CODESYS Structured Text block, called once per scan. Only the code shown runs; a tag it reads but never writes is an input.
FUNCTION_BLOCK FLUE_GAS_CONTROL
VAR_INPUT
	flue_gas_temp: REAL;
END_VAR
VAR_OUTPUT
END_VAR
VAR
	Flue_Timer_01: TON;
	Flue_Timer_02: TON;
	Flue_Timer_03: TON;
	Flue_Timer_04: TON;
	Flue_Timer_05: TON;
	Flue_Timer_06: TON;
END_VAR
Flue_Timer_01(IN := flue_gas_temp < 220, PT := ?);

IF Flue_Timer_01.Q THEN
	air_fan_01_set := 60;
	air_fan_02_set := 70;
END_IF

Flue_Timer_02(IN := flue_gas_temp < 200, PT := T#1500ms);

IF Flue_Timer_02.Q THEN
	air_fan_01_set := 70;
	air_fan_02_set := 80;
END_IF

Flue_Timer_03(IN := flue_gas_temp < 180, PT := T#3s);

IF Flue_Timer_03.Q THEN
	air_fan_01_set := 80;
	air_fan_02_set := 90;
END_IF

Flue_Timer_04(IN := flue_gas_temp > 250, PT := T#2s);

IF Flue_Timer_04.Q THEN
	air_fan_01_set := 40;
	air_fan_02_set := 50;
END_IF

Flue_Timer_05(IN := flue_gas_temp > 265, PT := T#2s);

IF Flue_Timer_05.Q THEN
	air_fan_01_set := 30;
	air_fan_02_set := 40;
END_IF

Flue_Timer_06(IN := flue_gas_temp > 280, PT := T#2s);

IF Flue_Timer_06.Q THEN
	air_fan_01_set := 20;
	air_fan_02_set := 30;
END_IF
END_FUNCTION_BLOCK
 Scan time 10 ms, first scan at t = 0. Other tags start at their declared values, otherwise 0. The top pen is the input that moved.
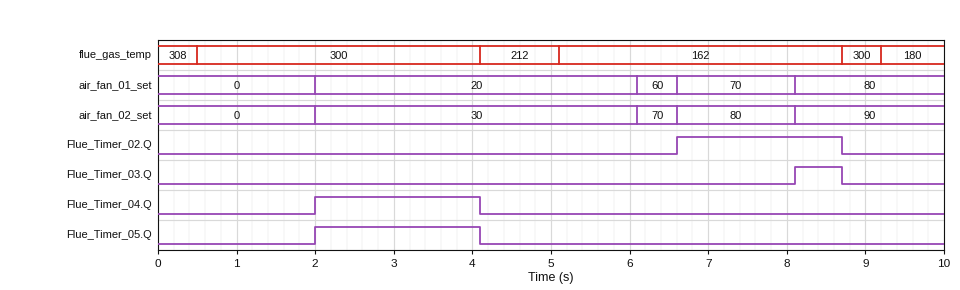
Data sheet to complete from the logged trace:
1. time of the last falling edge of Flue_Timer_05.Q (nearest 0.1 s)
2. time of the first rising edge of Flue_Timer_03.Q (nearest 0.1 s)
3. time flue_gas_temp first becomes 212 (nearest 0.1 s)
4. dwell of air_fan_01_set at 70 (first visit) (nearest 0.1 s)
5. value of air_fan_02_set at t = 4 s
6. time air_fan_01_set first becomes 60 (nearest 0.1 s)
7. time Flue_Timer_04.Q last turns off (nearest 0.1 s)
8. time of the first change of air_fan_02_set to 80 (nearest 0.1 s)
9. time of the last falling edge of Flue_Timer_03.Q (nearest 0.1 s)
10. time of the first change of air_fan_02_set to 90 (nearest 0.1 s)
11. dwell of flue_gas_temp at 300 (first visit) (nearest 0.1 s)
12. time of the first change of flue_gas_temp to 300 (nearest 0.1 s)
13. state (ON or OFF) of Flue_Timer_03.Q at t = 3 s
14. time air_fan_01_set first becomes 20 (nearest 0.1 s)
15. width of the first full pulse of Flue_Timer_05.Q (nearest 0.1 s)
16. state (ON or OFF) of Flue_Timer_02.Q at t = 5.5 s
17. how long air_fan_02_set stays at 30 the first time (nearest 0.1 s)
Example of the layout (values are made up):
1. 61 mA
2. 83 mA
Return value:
1. 4.1 s
2. 8.1 s
3. 4.1 s
4. 1.5 s
5. 30
6. 6.1 s
7. 4.1 s
8. 6.6 s
9. 8.7 s
10. 8.1 s
11. 3.6 s
12. 0.5 s
13. OFF
14. 2.0 s
15. 2.1 s
16. OFF
17. 4.1 s
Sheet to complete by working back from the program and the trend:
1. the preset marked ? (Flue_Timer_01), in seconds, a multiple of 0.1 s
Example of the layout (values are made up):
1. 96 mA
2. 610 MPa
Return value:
1. 2.0 s
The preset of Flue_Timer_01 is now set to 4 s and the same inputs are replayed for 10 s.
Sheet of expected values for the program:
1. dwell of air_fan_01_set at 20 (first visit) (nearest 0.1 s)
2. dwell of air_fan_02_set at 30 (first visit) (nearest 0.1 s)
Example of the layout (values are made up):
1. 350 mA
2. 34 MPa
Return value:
1. 4.6 s
2. 4.6 s
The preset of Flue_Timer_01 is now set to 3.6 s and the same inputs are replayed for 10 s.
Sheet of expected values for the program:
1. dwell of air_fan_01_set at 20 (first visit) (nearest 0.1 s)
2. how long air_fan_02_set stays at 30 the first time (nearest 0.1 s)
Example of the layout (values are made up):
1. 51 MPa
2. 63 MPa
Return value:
1. 4.6 s
2. 4.6 s
